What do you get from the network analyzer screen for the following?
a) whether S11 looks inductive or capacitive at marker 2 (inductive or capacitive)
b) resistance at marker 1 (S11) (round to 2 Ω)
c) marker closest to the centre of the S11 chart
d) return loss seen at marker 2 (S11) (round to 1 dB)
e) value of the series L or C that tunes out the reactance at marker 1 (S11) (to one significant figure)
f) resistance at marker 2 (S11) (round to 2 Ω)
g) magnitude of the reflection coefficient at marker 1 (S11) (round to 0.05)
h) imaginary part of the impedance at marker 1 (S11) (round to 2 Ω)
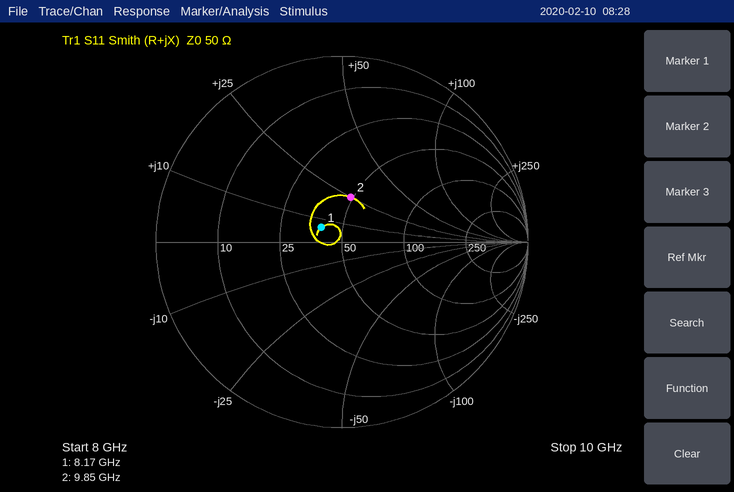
inductive
40 Ω
marker 1
12 dB
3 pF
48 Ω
0.15
+6 Ω
